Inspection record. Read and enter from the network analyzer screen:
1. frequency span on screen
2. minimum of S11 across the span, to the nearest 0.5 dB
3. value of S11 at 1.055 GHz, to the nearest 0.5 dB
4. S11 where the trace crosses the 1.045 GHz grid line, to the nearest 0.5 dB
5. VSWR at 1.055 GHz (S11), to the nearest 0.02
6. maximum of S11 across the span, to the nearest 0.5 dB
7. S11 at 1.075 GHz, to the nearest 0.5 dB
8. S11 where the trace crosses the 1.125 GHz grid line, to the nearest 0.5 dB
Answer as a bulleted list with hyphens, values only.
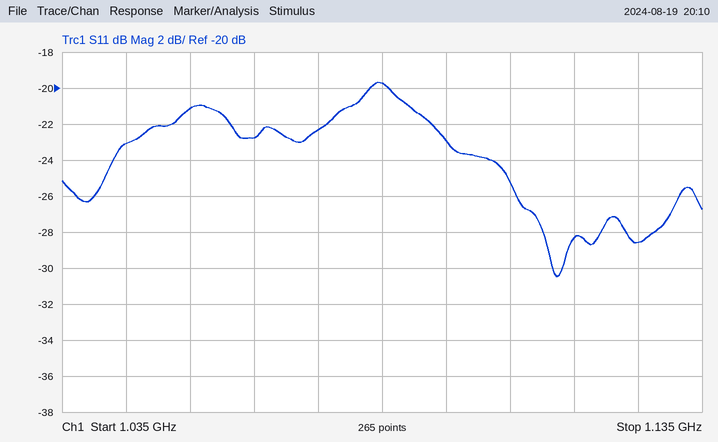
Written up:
- 100 MHz
- -30.5 dB
- -21.0 dB
- -23.0 dB
- 1.20
- -19.5 dB
- -22.5 dB
- -28.5 dB
